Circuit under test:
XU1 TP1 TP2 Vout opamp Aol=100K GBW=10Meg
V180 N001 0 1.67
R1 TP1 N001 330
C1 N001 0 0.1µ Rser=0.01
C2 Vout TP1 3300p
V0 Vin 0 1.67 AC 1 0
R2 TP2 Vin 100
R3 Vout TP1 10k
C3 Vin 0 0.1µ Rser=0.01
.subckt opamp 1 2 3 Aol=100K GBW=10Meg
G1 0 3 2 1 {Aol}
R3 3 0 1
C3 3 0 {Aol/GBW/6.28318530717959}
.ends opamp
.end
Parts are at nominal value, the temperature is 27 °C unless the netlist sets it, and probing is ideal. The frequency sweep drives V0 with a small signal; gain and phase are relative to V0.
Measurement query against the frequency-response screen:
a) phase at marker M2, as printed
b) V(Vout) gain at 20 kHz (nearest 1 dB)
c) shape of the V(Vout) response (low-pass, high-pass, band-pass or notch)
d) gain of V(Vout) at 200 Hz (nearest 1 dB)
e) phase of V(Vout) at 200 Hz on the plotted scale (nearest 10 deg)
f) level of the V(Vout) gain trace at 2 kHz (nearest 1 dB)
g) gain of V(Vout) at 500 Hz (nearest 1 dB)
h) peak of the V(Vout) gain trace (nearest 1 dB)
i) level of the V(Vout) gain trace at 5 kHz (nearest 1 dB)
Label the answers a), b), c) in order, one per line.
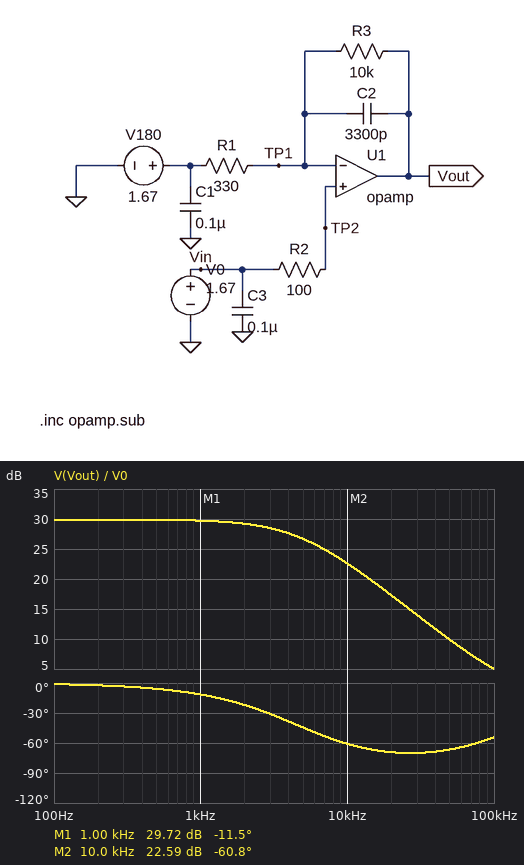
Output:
a) -60.8 deg
b) 17 dB
c) low-pass
d) 30 dB
e) 0 deg
f) 29 dB
g) 30 dB
h) 30 dB
i) 27 dB
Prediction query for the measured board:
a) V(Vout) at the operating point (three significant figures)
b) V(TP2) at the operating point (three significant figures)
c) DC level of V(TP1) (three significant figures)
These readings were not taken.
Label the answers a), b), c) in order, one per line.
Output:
a) 1.67 V
b) 1.67 V
c) 1.67 V
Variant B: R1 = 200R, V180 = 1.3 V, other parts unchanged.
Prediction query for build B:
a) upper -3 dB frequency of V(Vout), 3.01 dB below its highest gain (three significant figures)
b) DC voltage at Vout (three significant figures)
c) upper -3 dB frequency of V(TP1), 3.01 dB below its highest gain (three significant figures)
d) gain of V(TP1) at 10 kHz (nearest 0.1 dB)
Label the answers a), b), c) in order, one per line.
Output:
a) 4.71 kHz
b) 20.2 V
c) 9.76 MHz
d) -0.2 dB
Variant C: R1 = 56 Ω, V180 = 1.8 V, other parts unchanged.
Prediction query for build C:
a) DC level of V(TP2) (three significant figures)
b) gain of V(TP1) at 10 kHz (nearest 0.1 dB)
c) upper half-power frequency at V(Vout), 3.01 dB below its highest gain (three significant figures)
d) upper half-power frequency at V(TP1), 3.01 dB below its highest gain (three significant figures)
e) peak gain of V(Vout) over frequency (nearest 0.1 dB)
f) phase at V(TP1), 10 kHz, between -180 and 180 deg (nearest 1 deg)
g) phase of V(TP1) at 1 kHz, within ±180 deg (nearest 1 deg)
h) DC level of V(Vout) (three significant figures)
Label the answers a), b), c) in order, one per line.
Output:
a) 1.67 V
b) -0.6 dB
c) 4.45 kHz
d) 9.10 MHz
e) 45.1 dB
f) -2 deg
g) -1 deg
h) -21.5 V
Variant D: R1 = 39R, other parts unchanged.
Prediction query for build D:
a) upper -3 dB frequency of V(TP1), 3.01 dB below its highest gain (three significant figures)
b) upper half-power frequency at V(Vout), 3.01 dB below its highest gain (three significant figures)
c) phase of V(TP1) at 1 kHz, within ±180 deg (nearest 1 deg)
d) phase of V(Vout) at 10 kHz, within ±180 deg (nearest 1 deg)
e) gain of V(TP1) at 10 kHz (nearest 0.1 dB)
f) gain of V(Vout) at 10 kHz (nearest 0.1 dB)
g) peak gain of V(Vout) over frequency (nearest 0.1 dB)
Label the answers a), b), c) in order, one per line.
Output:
a) 8.65 MHz
b) 4.30 kHz
c) -1 deg
d) -66 deg
e) -0.8 dB
f) 40.1 dB
g) 48.2 dB
